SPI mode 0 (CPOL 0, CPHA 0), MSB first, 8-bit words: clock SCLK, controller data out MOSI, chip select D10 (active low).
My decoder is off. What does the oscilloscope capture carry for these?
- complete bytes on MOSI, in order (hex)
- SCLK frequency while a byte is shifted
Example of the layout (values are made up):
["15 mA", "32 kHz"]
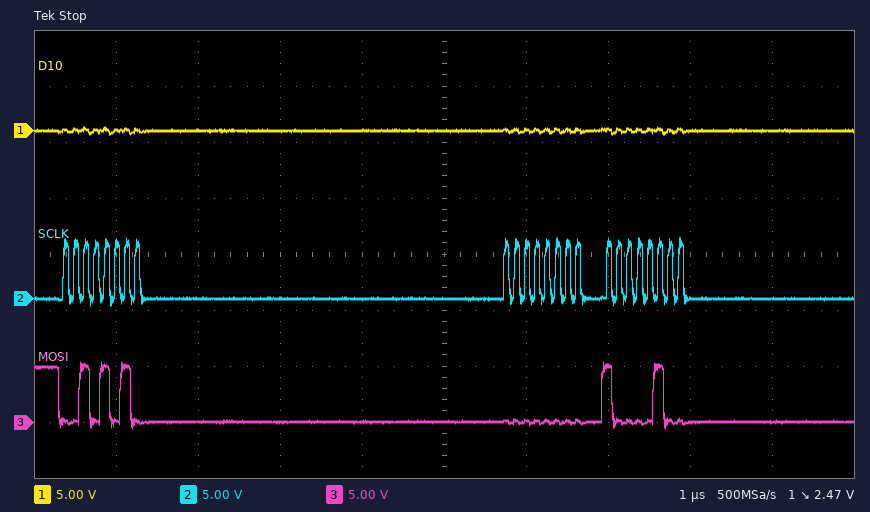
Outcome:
["0x2A 0x00 0x84", "8 MHz"]
